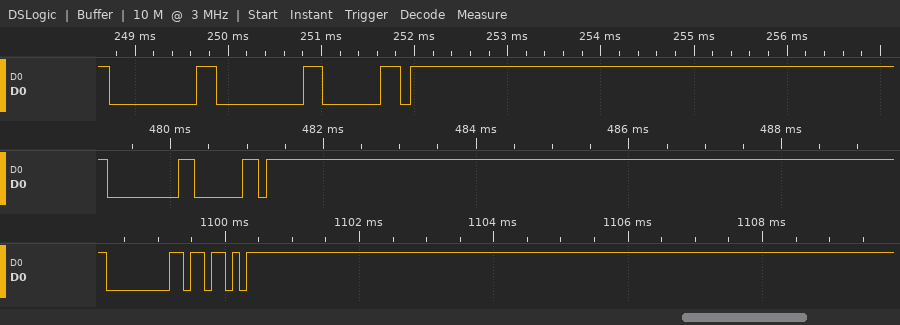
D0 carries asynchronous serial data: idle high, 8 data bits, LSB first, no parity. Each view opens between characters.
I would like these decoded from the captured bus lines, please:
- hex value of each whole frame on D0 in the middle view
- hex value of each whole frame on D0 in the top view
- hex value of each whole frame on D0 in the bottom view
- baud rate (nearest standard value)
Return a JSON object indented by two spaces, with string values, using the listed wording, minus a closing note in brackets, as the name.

{
  "hex value of each whole frame on D0 in the middle view": "00, 60",
  "hex value of each whole frame on D0 in the top view": "00, 00, 60",
  "hex value of each whole frame on D0 in the bottom view": "00, 5B",
  "baud rate": "9600 baud"
}
